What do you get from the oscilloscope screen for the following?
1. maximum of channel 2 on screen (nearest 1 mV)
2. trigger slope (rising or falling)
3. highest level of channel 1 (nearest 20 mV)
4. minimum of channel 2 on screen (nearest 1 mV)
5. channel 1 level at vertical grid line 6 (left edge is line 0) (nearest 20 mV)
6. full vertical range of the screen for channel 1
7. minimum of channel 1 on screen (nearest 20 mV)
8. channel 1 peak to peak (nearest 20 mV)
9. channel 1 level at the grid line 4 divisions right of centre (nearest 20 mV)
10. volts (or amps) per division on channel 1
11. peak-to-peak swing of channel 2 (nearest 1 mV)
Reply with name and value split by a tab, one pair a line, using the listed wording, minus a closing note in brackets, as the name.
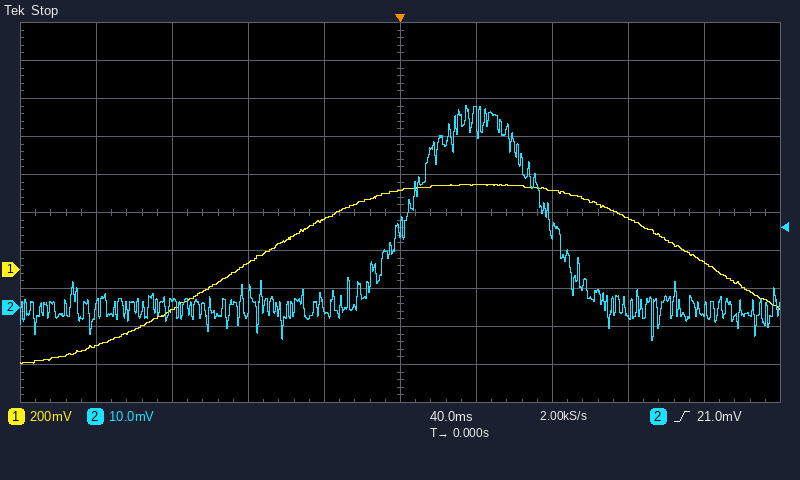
maximum of channel 2 on screen	53 mV
trigger slope	rising
highest level of channel 1	440 mV
minimum of channel 2 on screen	-9 mV
channel 1 level at vertical grid line 6 (left edge is line 0)	440 mV
full vertical range of the screen for channel 1	2 V
minimum of channel 1 on screen	-500 mV
channel 1 peak to peak	940 mV
channel 1 level at the grid line 4 divisions right of centre	40 mV
volts (or amps) per division on channel 1	200 mV
peak-to-peak swing of channel 2	62 mV
